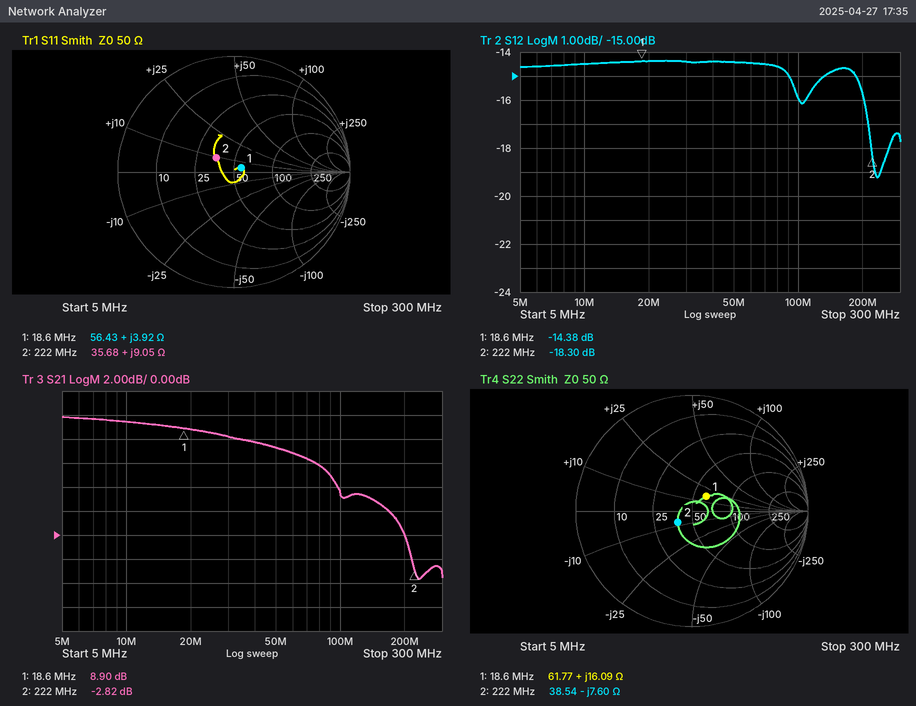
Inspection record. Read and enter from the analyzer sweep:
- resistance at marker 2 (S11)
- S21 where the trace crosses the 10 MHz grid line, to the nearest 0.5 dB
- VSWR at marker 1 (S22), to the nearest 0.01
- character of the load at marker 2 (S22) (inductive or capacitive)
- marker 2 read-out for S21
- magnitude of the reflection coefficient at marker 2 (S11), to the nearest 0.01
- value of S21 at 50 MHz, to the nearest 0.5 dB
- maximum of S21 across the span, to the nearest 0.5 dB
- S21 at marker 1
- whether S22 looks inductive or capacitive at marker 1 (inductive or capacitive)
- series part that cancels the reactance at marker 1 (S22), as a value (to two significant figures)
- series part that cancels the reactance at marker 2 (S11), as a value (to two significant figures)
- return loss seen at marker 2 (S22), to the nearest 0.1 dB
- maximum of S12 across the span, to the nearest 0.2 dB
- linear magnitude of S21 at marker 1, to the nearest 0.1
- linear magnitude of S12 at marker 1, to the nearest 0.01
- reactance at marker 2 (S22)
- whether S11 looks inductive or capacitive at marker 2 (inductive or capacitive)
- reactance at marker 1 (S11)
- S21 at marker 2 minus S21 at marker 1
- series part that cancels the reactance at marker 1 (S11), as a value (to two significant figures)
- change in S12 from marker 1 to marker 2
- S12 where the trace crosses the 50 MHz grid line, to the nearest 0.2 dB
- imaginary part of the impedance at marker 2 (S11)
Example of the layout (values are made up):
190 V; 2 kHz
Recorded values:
35.68 Ω; 9.5 dB; 1.43; capacitive; -2.82 dB; 0.20; 7.5 dB; 10.0 dB; 8.90 dB; inductive; 530 pF; 79 pF; 16.2 dB; -14.4 dB; 2.8; 0.19; -7.60 Ω; inductive; +3.92 Ω; -11.72 dB; 2.2 nF; -3.92 dB; -14.4 dB; +9.05 Ω
